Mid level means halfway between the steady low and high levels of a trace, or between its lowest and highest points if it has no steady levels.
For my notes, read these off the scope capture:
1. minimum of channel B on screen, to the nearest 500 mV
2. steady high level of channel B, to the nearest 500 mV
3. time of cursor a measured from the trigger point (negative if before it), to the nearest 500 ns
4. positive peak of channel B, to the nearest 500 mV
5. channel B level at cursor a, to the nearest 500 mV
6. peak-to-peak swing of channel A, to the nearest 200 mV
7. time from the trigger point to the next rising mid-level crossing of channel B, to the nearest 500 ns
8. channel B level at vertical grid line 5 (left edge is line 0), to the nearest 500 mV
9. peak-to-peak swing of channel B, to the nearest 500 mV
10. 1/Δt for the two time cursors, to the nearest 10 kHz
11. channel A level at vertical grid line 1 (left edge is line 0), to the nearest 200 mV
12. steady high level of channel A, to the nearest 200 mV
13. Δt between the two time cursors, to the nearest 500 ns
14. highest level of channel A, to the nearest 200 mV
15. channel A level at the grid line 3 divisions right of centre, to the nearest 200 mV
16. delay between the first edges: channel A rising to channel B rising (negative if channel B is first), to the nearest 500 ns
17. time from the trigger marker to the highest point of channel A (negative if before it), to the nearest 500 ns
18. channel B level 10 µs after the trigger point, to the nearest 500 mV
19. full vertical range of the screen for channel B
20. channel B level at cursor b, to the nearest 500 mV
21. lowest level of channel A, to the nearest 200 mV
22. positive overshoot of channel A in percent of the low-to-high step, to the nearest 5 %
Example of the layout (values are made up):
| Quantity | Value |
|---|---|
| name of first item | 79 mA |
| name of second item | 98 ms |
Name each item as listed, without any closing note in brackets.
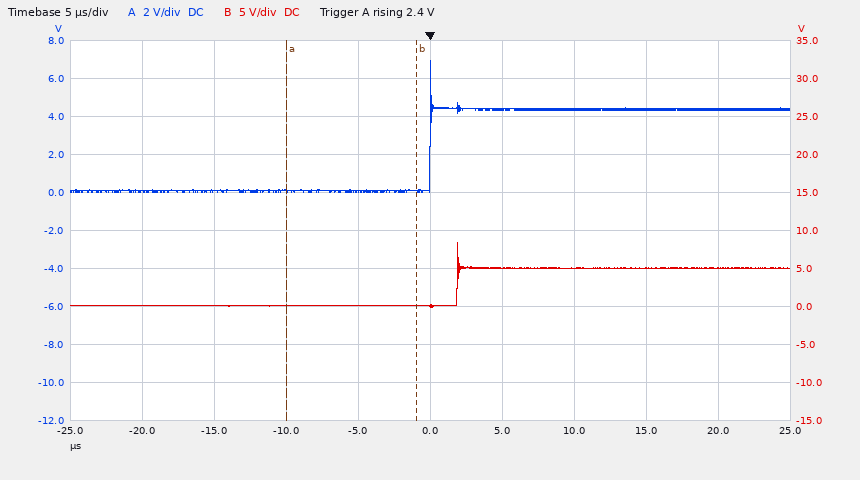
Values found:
| Quantity | Value |
|---|---|
| minimum of channel B on screen, to the nearest 500 mV | 0.0 V |
| steady high level of channel B, to the nearest 500 mV | 5.0 V |
| time of cursor a measured from the trigger point (negative if before it), to the nearest 500 ns | -10.0 µs |
| positive peak of channel B, to the nearest 500 mV | 8.5 V |
| channel B level at cursor a, to the nearest 500 mV | 0.0 V |
| peak-to-peak swing of channel A, to the nearest 200 mV | 7.0 V |
| time from the trigger point to the next rising mid-level crossing of channel B, to the nearest 500 ns | 2.0 µs |
| channel B level at vertical grid line 5 (left edge is line 0), to the nearest 500 mV | 0.0 V |
| peak-to-peak swing of channel B, to the nearest 500 mV | 8.5 V |
| 1/Δt for the two time cursors, to the nearest 10 kHz | 110 kHz |
| channel A level at vertical grid line 1 (left edge is line 0), to the nearest 200 mV | 0.0 V |
| steady high level of channel A, to the nearest 200 mV | 4.4 V |
| Δt between the two time cursors, to the nearest 500 ns | 9.0 µs |
| highest level of channel A, to the nearest 200 mV | 7.0 V |
| channel A level at the grid line 3 divisions right of centre, to the nearest 200 mV | 4.4 V |
| delay between the first edges: channel A rising to channel B rising (negative if channel B is first), to the nearest 500 ns | +2.0 µs |
| time from the trigger marker to the highest point of channel A (negative if before it), to the nearest 500 ns | 0.0 µs |
| channel B level 10 µs after the trigger point, to the nearest 500 mV | 5.0 V |
| full vertical range of the screen for channel B | 50 V |
| channel B level at cursor b, to the nearest 500 mV | 0.0 V |
| lowest level of channel A, to the nearest 200 mV | 0.0 V |
| positive overshoot of channel A in percent of the low-to-high step, to the nearest 5 % | 60 % |
